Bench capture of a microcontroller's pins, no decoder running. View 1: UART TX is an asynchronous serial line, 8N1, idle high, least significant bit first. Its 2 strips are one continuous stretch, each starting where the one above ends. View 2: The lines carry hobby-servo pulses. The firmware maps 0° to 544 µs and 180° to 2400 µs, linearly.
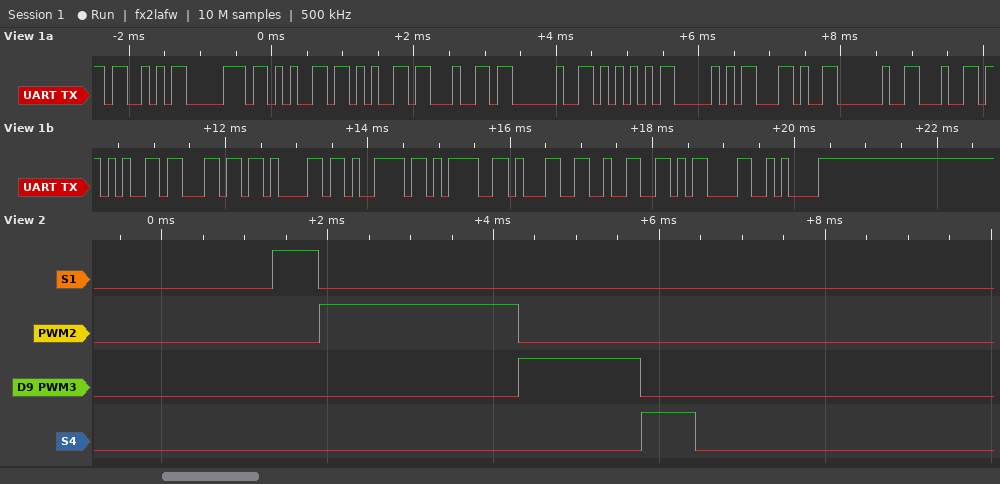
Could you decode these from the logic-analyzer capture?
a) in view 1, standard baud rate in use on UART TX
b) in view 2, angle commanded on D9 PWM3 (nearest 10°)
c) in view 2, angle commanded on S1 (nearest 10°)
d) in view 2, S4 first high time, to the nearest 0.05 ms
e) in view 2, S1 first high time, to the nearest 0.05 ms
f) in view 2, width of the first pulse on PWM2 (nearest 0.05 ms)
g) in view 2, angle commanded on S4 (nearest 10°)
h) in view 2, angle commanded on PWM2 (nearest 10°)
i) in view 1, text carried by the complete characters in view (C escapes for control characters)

9600 baud
90°
0°
0.65 ms
0.55 ms
2.40 ms
10°
180°
"Speed UP, delay=12\r\n"
